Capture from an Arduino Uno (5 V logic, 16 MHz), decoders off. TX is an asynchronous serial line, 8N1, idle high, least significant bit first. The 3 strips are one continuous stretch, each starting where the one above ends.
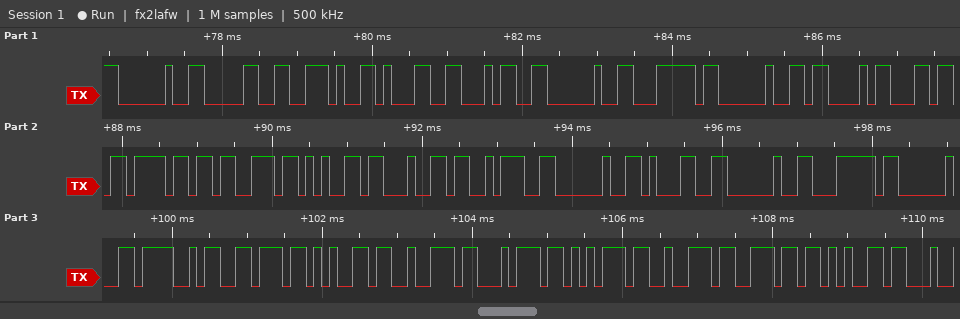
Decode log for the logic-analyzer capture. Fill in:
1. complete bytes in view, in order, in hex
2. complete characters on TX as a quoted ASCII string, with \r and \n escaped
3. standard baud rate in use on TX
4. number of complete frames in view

20 30 2E 31 34 20 7C 20 43 6C 6F 73 65 64 3A 20 31 20 7C 20 4F 76 65 72 74 75 72 6E 65
" 0.14 | Closed: 1 | Overturne"
9600 baud
29
